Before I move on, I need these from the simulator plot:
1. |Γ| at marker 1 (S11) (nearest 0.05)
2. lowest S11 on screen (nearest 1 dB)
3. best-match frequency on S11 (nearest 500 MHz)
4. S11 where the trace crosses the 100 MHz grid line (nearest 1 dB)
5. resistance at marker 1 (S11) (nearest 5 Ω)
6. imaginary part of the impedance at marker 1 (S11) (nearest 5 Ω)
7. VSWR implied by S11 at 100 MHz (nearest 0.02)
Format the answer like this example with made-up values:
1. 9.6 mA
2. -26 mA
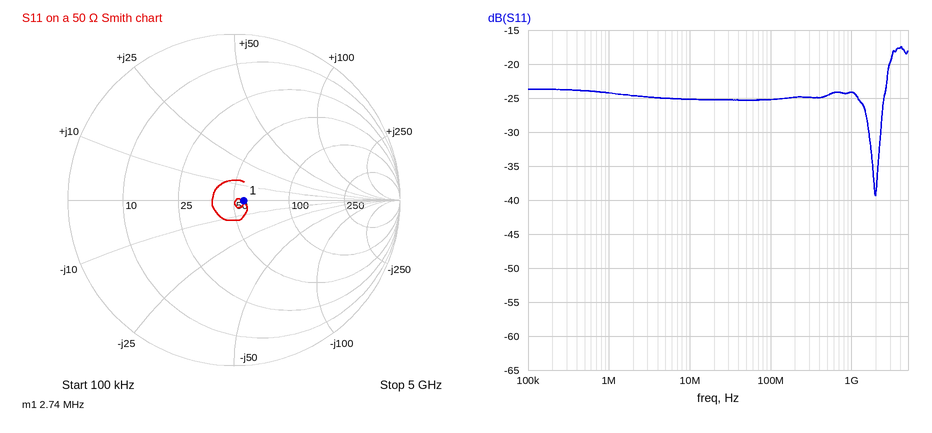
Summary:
1. 0.05
2. -39 dB
3. 2.0 GHz
4. -25 dB
5. 55 Ω
6. 0 Ω
7. 1.12
